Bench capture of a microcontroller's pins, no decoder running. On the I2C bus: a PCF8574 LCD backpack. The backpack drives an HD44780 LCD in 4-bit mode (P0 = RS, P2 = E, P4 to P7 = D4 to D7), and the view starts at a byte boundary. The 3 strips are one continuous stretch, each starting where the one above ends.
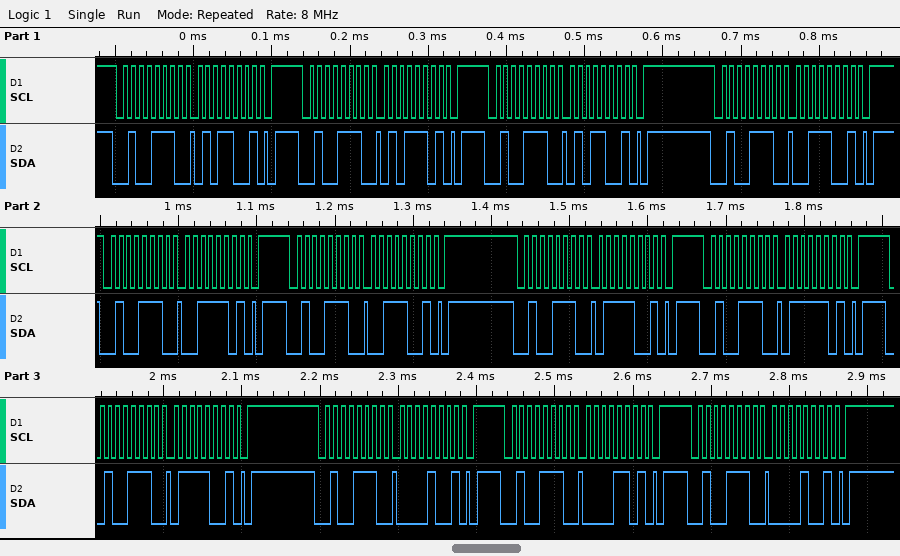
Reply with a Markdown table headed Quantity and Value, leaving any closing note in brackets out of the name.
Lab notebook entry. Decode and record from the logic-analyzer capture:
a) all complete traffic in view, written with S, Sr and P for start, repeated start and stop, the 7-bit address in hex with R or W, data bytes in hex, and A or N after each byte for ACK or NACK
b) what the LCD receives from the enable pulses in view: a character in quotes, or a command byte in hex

| Quantity | Value |
|---|---|
| all complete traffic in view, written with S, Sr and P for start, repeated start and stop, the 7-bit address in hex with R or W, data bytes in hex, and A or N after each byte for ACK or NACK | S 27W A 59 A P S 27W A 5D A P S 27W A 59 A P S 27W A 39 A P S 27W A 3D A P S 27W A 39 A P S 27W A 79 A P S 27W A 7D A P S 27W A 79 A P S 27W A 09 A P S 27W A 0D A P S 27W A 09 A P |
| what the LCD receives from the enable pulses in view: a character in quotes, or a command byte in hex | 'S' 'p' |
